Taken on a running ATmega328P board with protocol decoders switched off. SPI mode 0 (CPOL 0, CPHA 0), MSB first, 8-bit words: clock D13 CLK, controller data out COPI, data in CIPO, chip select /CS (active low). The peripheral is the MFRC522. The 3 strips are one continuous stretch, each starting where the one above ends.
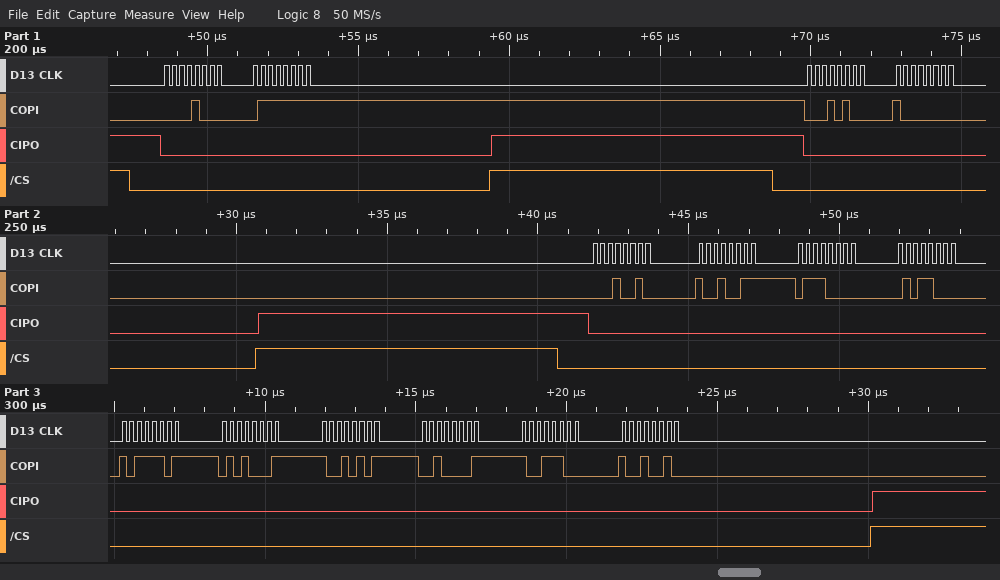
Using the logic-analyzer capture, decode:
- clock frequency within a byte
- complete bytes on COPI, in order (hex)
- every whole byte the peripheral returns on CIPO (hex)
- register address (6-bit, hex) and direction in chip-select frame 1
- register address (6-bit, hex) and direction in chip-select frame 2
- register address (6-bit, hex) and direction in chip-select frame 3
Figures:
4 MHz
0x08 0x7F 0x14 0x80 0x12 0x93 0x70 0x58 0xBD 0x51 0x95 0x21 0x9C 0x92
0x00 0x00 0x00 0x00 0x00 0x00 0x00 0x00 0x00 0x00 0x00 0x00 0x00 0x00
0x04 write
0x0A write
0x09 write
